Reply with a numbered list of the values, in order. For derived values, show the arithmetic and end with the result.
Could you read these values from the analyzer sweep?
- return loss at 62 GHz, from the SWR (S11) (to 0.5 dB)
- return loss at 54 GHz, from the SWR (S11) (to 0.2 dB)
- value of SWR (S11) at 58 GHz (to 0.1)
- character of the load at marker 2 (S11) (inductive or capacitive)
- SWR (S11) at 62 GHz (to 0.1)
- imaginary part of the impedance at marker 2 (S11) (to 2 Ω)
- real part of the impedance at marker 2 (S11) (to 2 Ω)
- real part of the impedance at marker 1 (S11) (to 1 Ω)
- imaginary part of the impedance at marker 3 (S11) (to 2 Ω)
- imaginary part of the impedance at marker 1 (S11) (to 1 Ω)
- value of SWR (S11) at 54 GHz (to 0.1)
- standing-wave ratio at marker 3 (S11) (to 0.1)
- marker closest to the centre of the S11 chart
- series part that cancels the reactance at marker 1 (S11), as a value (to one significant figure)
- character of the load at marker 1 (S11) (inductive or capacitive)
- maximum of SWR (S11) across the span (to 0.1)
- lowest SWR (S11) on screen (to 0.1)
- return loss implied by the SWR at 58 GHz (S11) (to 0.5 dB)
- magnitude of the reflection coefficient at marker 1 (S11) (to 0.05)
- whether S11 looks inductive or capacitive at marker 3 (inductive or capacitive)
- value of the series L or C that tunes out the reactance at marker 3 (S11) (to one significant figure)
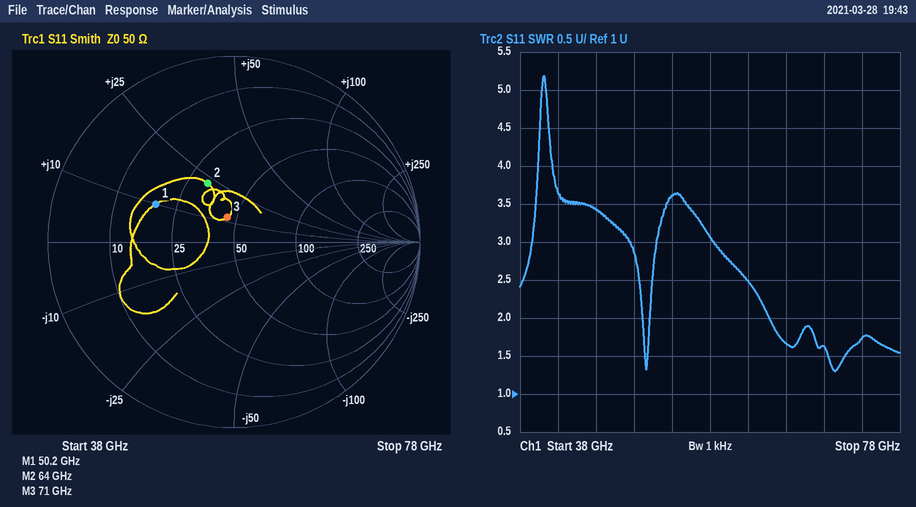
1. −20 log10((2.5 − 1)/(2.5 + 1)) ≈ 7.36 dB, so 7.5 dB to the nearest 0.5 dB
2. −20 log10((3.6 − 1)/(3.6 + 1)) ≈ 5.0 dB
3. 3.1
4. inductive
5. 2.5
6. +22 Ω
7. 32 Ω
8. 19 Ω
9. +12 Ω
10. +10 Ω
11. 3.6
12. 1.3
13. marker 3
14. C = 1/(2π × 50.2 GHz × 10 Ω) ≈ 317 fF, so 300 fF to one significant figure
15. inductive
16. 5.2
17. 1.3
18. −20 log10((3.1 − 1)/(3.1 + 1)) ≈ 5.81 dB, so 6.0 dB to the nearest 0.5 dB
19. 0.45
20. inductive
21. C = 1/(2π × 71 GHz × 12 Ω) ≈ 187 fF, so 200 fF to one significant figure
